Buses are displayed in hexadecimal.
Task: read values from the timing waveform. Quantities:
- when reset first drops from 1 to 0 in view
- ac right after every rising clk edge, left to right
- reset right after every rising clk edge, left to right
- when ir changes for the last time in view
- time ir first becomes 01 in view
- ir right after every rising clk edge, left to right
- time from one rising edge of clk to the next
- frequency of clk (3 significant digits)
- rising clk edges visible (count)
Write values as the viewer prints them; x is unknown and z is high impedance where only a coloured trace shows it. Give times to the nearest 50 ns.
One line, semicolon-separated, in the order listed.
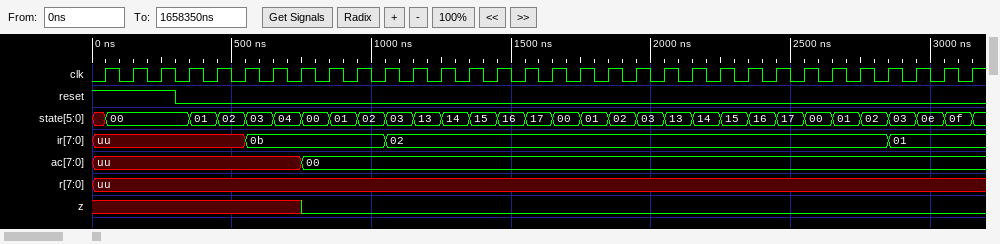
300 ns; uu, uu, uu, uu, uu, uu, uu, 00, 00, 00, 00, 00, 00, 00, 00, 00, 00, 00, 00, 00, 00, 00, 00, 00, 00, 00, 00, 00, 00, 00, 00, 00; 1 1 1 0 0 0 0 0 0 0 0 0 0 0 0 0 0 0 0 0 0 0 0 0 0 0 0 0 0 0 0 0; 2850 ns; 2850 ns; uu, uu, uu, uu, uu, 0b, 0b, 0b, 0b, 0b, 02, 02, 02, 02, 02, 02, 02, 02, 02, 02, 02, 02, 02, 02, 02, 02, 02, 02, 01, 01, 01, 01; 100 ns; 10.0 MHz; 32
